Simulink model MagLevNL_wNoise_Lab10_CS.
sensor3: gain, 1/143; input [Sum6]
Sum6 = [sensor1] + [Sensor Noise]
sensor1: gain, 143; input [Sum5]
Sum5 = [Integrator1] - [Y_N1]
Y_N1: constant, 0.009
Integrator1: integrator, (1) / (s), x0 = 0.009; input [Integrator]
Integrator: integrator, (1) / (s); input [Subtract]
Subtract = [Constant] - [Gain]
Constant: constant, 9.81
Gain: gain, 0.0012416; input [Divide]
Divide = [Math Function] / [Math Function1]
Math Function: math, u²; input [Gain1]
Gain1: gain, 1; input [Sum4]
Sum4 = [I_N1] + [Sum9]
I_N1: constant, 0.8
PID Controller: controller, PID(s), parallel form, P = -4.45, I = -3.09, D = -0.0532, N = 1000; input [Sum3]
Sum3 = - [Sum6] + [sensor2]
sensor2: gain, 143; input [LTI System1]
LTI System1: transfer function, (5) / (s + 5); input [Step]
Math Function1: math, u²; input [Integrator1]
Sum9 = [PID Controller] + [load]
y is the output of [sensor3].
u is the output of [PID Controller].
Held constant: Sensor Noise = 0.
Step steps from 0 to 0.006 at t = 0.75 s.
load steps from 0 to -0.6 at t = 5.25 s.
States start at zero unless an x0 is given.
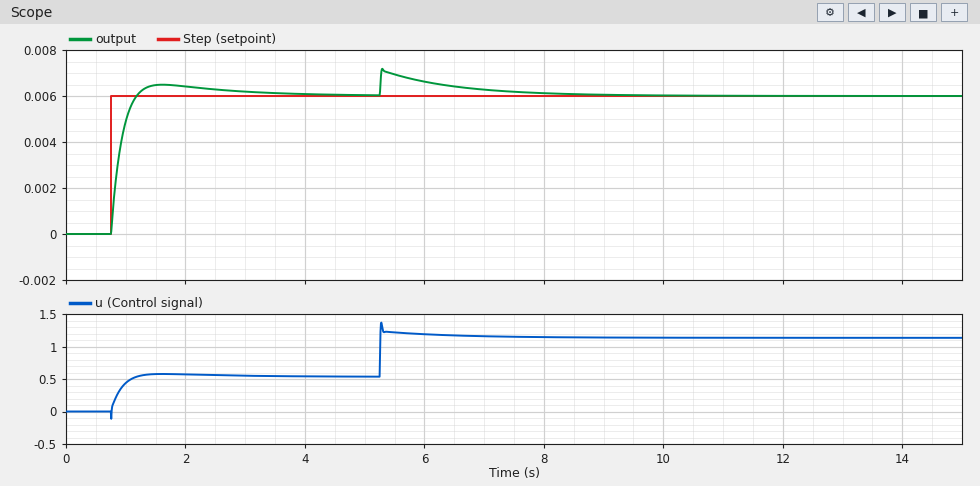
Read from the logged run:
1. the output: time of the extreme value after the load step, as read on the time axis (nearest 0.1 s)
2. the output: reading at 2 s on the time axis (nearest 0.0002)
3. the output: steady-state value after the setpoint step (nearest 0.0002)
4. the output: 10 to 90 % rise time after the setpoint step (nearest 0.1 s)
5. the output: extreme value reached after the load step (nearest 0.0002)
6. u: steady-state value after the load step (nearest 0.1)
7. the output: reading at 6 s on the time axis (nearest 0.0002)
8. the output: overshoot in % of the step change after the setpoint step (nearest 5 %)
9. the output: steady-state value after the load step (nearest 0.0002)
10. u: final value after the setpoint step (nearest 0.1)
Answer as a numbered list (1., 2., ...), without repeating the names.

1. 5.3 s
2. 0.0064
3. 0.0060
4. 0.3 s
5. 0.0072
6. 1.1
7. 0.0066
8. 10 %
9. 0.0060
10. 0.5
